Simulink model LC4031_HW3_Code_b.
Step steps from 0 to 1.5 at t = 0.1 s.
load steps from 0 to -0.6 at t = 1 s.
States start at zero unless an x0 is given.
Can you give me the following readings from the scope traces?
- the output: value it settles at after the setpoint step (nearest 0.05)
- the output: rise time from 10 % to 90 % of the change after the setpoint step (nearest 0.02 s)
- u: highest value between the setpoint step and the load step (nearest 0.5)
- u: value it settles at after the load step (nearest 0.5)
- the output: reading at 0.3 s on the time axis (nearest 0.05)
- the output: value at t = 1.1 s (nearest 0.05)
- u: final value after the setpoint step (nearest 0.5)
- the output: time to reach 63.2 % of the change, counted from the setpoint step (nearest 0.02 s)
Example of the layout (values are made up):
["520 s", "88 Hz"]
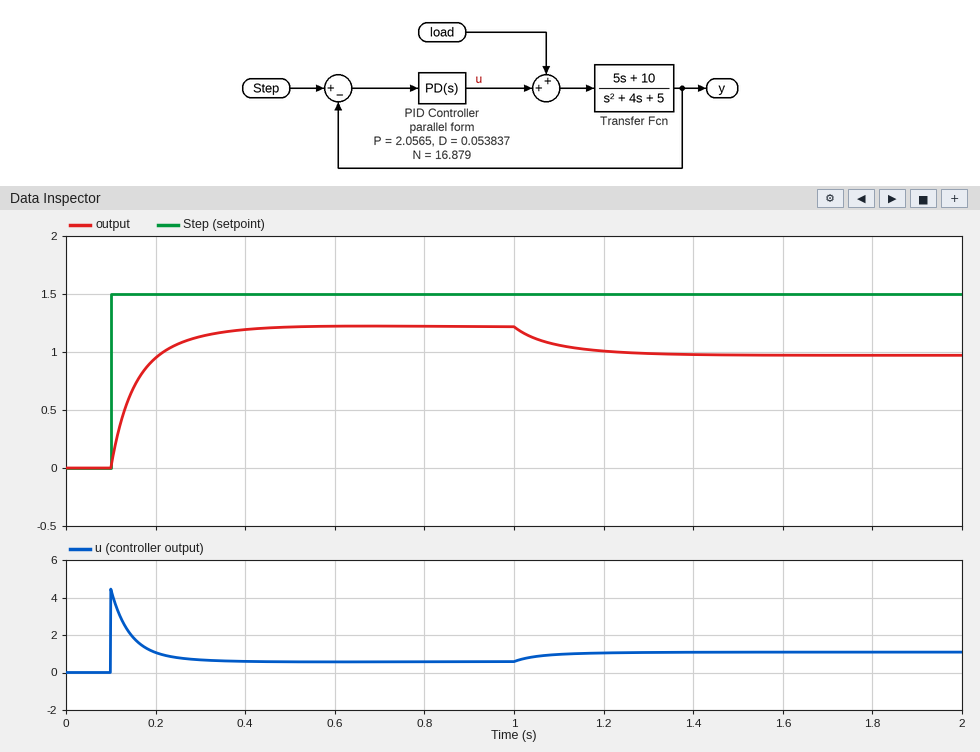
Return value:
["1.20", "0.16 s", "4.5", "1.0", "1.15", "1.05", "0.5", "0.06 s"]
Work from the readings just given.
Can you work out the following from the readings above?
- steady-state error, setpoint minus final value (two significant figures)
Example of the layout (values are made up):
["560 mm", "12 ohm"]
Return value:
["0.30"]
